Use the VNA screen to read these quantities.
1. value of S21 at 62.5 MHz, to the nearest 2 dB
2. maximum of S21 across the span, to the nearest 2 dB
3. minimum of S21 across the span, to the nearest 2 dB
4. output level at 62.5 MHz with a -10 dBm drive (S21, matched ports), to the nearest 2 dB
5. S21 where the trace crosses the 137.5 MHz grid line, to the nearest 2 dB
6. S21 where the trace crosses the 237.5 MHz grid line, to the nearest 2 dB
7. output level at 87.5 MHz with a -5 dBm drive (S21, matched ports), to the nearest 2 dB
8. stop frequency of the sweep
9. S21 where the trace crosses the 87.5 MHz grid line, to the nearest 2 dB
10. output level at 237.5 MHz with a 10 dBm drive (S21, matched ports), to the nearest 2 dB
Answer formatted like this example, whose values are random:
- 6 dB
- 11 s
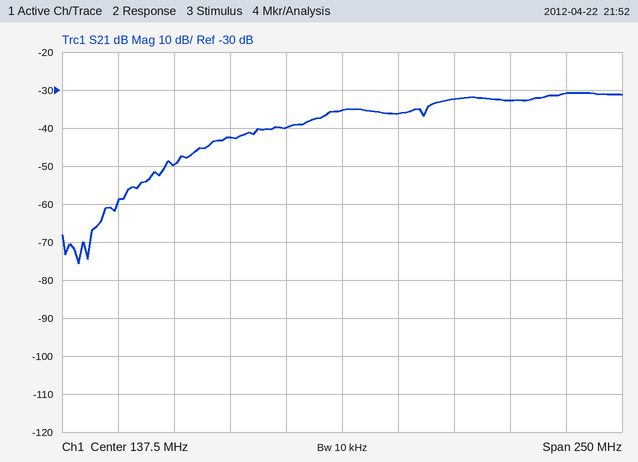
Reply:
- -50 dB
- -30 dB
- -76 dB
- -60 dBm
- -36 dB
- -30 dB
- -48 dBm
- 262.5 MHz
- -42 dB
- -20 dBm
